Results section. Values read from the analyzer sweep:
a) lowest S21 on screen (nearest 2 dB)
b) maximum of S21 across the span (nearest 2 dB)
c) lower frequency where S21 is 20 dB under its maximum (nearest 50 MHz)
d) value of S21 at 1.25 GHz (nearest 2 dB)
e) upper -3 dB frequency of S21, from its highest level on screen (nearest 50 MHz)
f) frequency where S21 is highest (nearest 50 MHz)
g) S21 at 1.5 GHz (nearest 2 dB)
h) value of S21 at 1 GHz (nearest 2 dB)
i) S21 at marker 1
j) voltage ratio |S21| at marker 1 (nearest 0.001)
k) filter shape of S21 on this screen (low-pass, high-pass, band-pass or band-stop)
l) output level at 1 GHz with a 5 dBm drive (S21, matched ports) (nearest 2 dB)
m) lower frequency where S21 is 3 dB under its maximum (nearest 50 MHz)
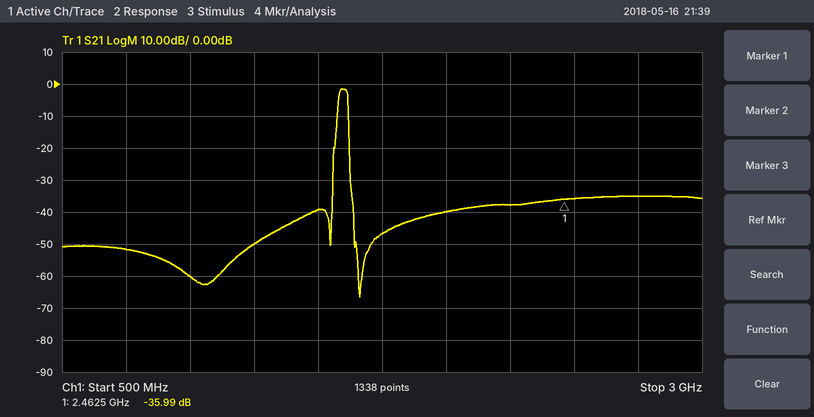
-66 dB
-2 dB
1.55 GHz
-50 dB
1.60 GHz
1.60 GHz
-40 dB
-60 dB
-35.99 dB
0.016
band-pass
-56 dBm
1.60 GHz
